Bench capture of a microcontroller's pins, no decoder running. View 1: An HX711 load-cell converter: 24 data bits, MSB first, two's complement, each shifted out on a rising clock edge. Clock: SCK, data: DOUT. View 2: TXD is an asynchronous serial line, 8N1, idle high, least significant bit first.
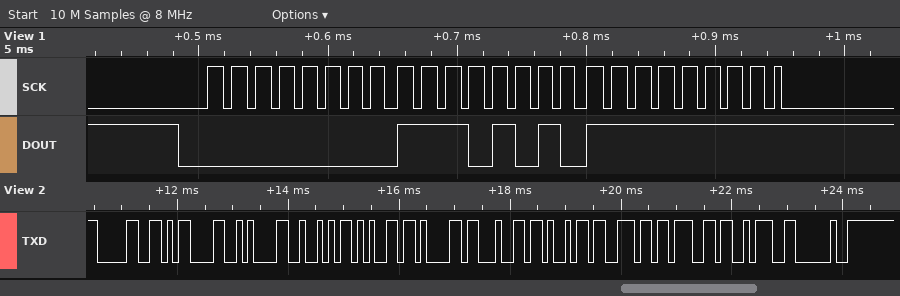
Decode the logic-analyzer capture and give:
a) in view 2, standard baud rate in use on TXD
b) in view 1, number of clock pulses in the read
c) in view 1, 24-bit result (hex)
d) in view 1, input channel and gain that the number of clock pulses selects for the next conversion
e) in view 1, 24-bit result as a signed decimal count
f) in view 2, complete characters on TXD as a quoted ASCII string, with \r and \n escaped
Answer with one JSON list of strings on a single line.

["9600 baud", "25", "0x00EAFF", "channel A, gain 128", "60159", "\"0\\r\\nReading: \""]
